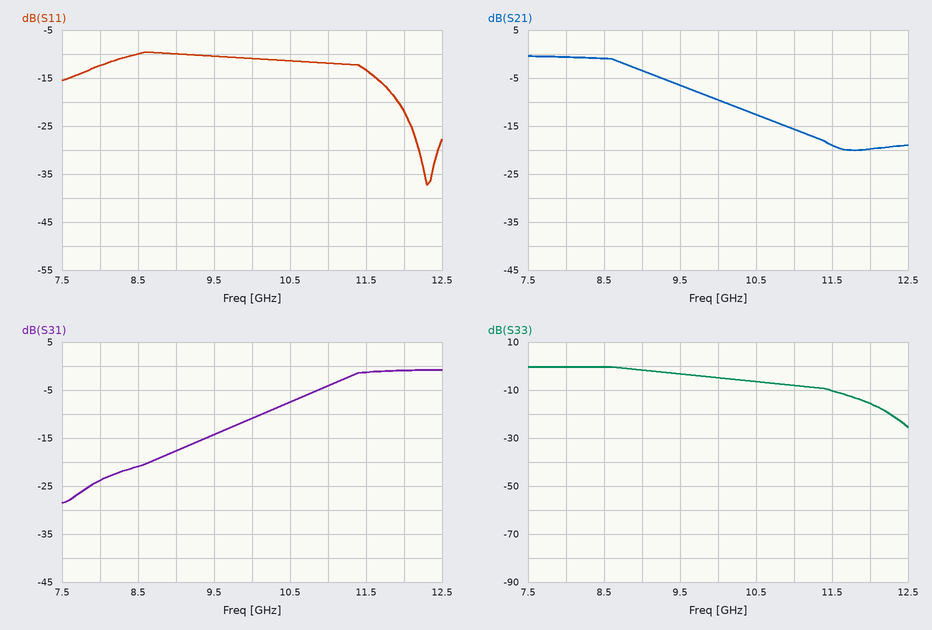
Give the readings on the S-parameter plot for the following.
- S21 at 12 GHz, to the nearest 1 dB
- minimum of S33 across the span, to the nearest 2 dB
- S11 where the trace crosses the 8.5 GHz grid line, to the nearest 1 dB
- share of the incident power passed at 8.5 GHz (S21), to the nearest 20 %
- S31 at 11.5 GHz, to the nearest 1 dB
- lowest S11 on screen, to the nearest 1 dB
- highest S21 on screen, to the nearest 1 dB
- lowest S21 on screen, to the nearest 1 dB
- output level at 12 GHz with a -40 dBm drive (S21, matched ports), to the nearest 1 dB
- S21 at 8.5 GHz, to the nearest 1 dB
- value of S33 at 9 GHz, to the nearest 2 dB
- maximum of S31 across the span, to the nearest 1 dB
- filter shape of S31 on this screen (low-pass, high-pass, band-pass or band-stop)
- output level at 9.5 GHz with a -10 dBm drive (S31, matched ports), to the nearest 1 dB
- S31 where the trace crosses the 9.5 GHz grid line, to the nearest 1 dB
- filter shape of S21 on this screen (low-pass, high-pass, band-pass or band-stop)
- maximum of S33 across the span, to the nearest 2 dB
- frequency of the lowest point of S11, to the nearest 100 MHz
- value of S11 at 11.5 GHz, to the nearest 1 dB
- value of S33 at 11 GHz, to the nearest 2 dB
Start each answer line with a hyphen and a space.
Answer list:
- -20 dB
- -26 dB
- -10 dB
- 80 %
- -1 dB
- -37 dB
- 0 dB
- -20 dB
- -60 dBm
- -1 dB
- -2 dB
- -1 dB
- high-pass
- -24 dBm
- -14 dB
- low-pass
- 0 dB
- 12.3 GHz
- -13 dB
- -8 dB
